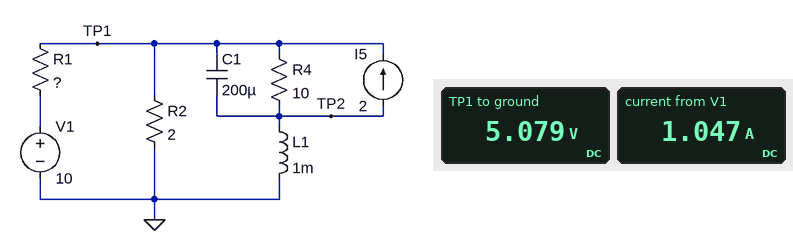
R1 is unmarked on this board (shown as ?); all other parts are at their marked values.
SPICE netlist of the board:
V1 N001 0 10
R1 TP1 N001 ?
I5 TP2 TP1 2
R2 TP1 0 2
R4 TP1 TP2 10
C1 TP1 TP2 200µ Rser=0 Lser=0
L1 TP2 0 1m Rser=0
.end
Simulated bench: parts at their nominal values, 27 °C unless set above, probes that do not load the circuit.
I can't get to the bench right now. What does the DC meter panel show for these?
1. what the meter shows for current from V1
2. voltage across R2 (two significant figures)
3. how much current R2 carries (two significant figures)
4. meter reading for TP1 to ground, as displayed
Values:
1.047 A
5.1 V
2.5 A
5.079 V
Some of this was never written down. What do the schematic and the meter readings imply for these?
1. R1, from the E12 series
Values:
4.7 Ω
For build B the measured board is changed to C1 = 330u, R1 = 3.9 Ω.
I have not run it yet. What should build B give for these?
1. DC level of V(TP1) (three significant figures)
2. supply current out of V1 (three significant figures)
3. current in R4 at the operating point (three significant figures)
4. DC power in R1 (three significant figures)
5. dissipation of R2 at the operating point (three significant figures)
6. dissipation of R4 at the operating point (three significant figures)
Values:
5.33 V
1.20 A
533 mA
5.59 W
14.2 W
2.84 W
